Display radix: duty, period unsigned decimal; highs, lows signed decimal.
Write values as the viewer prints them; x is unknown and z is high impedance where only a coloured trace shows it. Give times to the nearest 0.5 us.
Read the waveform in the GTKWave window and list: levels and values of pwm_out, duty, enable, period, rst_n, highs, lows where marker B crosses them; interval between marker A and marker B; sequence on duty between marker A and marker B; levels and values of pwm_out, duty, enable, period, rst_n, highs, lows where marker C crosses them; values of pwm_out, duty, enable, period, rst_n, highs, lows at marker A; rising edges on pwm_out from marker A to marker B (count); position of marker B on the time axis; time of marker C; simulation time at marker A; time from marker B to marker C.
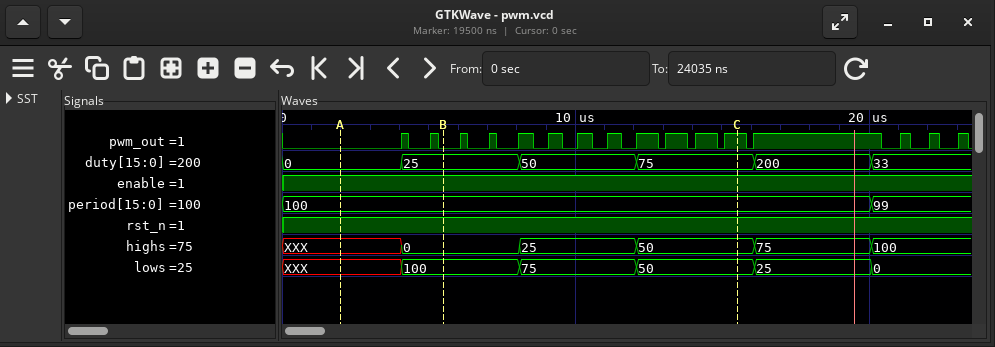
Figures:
pwm_out=0, duty=25, enable=1, period=100, rst_n=1, highs=0, lows=100
3.5 us
0, 25
pwm_out=1, duty=75, enable=1, period=100, rst_n=1, highs=50, lows=50
pwm_out=0, duty=0, enable=1, period=100, rst_n=1, highs=XXX, lows=XXX
2
5.5 us
15.5 us
2 us
10 us
